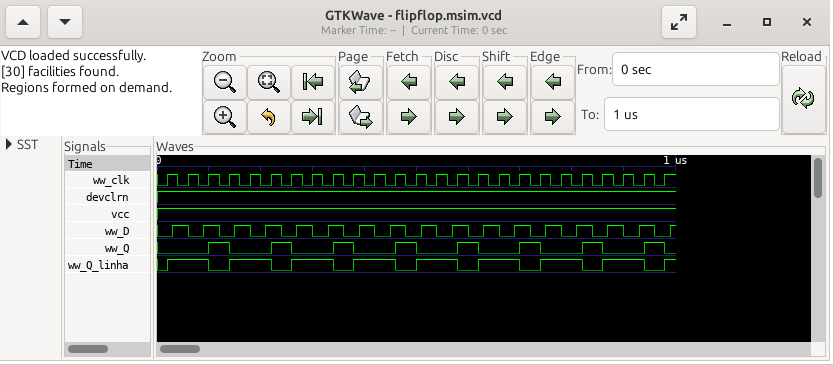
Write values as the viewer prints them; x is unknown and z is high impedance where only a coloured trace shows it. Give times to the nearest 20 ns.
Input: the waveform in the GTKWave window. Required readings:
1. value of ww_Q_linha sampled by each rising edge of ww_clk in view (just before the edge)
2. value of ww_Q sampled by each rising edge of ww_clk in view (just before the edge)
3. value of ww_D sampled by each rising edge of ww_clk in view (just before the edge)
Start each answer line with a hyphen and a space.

- 0 1 1 0 1 1 0 1 1 0 1 1 0 1 1 0 1 1 0 1 1 0 1 1 0
- 0 0 0 1 0 0 1 0 0 1 0 0 1 0 0 1 0 0 1 0 0 1 0 0 1
- 0 1 1 0 1 1 0 1 1 0 1 1 0 1 1 0 1 1 0 1 1 0 1 1 0
